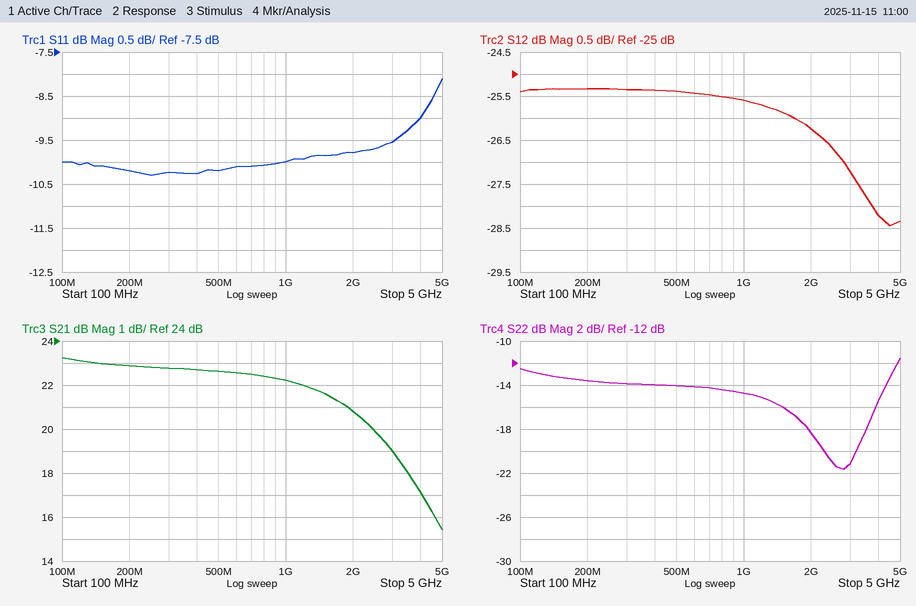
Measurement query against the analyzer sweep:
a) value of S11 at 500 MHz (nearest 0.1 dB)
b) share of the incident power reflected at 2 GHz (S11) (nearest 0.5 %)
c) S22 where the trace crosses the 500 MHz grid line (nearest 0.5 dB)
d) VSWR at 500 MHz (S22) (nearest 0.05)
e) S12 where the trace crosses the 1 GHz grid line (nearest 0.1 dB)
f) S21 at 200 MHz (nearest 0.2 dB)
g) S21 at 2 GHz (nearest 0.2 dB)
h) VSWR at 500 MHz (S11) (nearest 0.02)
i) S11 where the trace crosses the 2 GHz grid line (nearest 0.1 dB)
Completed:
-10.2 dB
10.5 %
-14.0 dB
1.50
-25.6 dB
22.8 dB
20.8 dB
1.90
-9.8 dB
